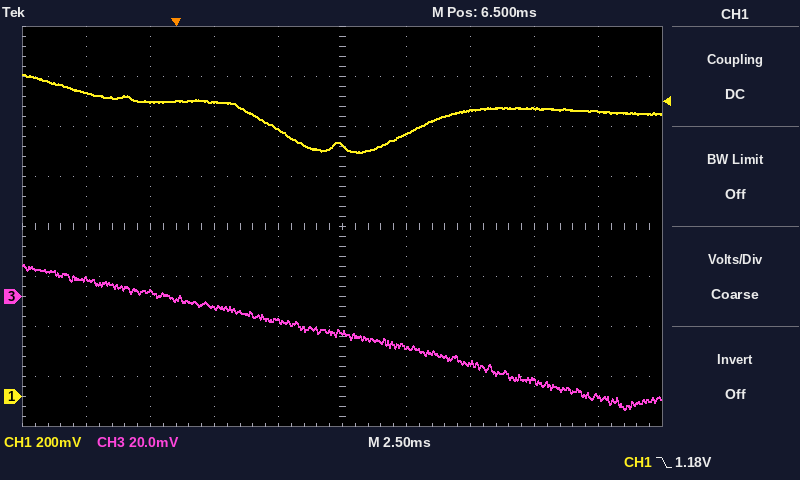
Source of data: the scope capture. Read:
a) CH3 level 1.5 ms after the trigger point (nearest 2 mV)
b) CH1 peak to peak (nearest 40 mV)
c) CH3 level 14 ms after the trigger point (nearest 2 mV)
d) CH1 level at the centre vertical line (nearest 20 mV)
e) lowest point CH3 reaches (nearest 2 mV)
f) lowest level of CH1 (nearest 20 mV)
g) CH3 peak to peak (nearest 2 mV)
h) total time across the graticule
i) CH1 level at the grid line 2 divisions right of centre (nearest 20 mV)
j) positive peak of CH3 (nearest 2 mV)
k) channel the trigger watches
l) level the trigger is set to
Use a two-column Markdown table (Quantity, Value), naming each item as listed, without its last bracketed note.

| Quantity | Value |
|---|---|
| CH3 level 1.5 ms after the trigger point | -4 mV |
| CH1 peak to peak | 320 mV |
| CH3 level 14 ms after the trigger point | -34 mV |
| CH1 level at the centre vertical line | 1.00 V |
| lowest point CH3 reaches | -46 mV |
| lowest level of CH1 | 980 mV |
| CH3 peak to peak | 58 mV |
| total time across the graticule | 25 ms |
| CH1 level at the grid line 2 divisions right of centre | 1.14 V |
| positive peak of CH3 | 12 mV |
| channel the trigger watches | CH1 |
| level the trigger is set to | 1.18 V |
